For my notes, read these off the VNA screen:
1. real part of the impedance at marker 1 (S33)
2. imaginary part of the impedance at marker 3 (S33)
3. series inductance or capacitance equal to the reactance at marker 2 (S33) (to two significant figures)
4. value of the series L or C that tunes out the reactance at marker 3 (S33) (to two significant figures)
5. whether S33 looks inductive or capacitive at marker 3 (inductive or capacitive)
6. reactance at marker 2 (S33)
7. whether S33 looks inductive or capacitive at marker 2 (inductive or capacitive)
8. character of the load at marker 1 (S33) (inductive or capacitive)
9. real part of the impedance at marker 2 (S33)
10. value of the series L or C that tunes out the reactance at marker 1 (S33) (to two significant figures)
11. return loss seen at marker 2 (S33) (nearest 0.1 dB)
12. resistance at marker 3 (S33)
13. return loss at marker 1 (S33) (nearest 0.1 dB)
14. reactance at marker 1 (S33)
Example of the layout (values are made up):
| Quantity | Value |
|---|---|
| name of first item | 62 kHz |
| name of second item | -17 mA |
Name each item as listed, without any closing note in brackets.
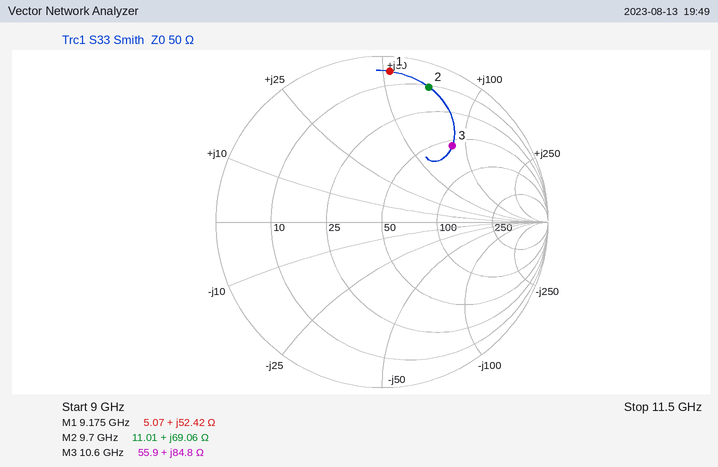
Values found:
| Quantity | Value |
|---|---|
| real part of the impedance at marker 1 | 5.07 Ω |
| imaginary part of the impedance at marker 3 | +84.8 Ω |
| series inductance or capacitance equal to the reactance at marker 2 (S33) | 1.1 nH |
| value of the series L or C that tunes out the reactance at marker 3 (S33) | 180 fF |
| whether S33 looks inductive or capacitive at marker 3 | inductive |
| reactance at marker 2 | +69.06 Ω |
| whether S33 looks inductive or capacitive at marker 2 | inductive |
| character of the load at marker 1 (S33) | inductive |
| real part of the impedance at marker 2 | 11.01 Ω |
| value of the series L or C that tunes out the reactance at marker 1 (S33) | 330 fF |
| return loss seen at marker 2 (S33) | 1.3 dB |
| resistance at marker 3 | 55.9 Ω |
| return loss at marker 1 (S33) | 0.8 dB |
| reactance at marker 1 | +52.42 Ω |
